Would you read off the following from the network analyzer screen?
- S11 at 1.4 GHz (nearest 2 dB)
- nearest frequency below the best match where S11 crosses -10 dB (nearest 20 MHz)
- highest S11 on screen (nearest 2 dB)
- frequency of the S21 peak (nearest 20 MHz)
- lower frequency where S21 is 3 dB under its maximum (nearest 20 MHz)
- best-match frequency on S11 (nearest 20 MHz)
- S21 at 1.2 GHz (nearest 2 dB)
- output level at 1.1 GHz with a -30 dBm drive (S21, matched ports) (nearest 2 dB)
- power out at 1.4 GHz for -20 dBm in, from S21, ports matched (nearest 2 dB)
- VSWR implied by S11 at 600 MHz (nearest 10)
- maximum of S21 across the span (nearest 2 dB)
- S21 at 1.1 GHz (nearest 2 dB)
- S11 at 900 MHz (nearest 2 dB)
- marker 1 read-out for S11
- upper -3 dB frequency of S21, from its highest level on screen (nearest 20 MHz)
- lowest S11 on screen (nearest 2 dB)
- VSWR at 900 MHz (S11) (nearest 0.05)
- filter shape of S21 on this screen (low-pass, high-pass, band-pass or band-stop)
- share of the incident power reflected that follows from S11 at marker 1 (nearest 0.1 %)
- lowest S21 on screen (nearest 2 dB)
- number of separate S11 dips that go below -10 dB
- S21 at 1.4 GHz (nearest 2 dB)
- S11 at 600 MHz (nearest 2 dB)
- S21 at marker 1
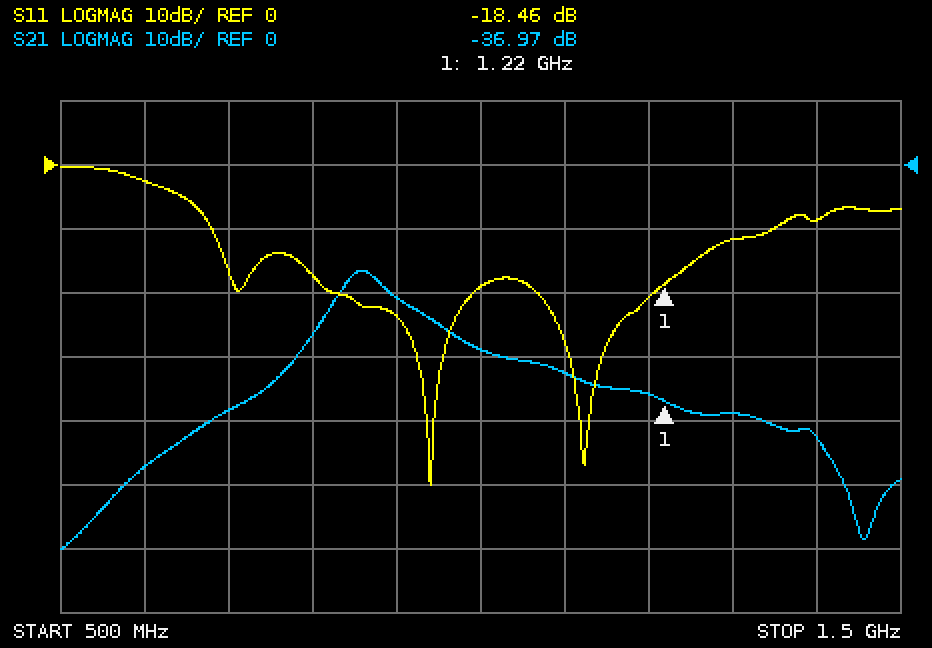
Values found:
-8 dB
680 MHz
0 dB
860 MHz
840 MHz
940 MHz
-36 dB
-62 dBm
-62 dBm
10
-16 dB
-32 dB
-24 dB
-18.46 dB
880 MHz
-50 dB
1.15
band-pass
1.4 %
-60 dB
3
-42 dB
-2 dB
-36.97 dB
